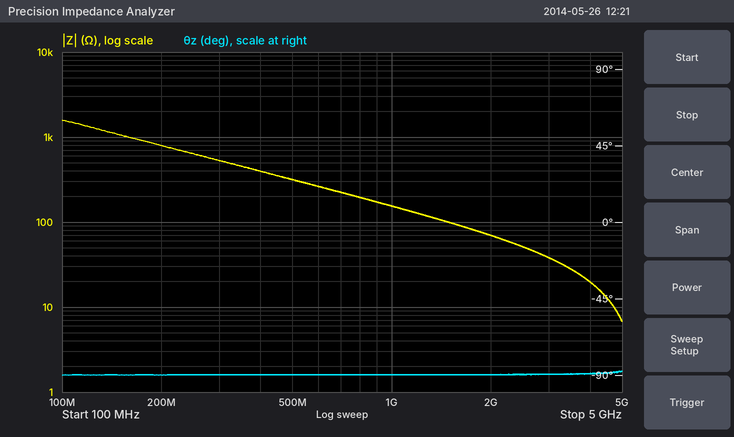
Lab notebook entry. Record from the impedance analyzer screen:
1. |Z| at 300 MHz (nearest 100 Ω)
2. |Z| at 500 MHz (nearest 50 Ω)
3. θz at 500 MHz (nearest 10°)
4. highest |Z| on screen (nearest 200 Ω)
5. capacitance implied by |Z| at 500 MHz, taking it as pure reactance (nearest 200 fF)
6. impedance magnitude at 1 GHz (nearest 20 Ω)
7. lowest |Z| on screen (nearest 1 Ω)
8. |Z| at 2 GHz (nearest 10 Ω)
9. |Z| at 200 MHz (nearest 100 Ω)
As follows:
500 Ω
300 Ω
-90°
1.6 kΩ
1.0 pF
160 Ω
7 Ω
70 Ω
800 Ω
